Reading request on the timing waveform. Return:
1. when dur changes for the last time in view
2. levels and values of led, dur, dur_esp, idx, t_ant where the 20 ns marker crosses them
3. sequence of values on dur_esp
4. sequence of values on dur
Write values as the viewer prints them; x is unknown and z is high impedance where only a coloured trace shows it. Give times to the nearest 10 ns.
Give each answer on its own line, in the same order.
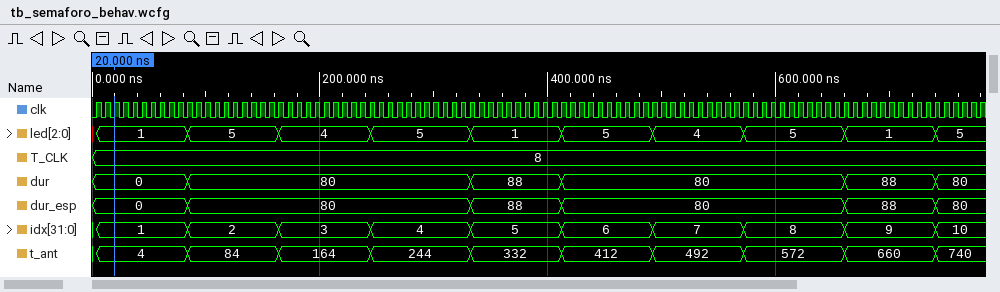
740 ns
led=1, dur=0, dur_esp=0, idx=1, t_ant=4
0, 80, 88, 80, 88, 80
0, 80, 88, 80, 88, 80
